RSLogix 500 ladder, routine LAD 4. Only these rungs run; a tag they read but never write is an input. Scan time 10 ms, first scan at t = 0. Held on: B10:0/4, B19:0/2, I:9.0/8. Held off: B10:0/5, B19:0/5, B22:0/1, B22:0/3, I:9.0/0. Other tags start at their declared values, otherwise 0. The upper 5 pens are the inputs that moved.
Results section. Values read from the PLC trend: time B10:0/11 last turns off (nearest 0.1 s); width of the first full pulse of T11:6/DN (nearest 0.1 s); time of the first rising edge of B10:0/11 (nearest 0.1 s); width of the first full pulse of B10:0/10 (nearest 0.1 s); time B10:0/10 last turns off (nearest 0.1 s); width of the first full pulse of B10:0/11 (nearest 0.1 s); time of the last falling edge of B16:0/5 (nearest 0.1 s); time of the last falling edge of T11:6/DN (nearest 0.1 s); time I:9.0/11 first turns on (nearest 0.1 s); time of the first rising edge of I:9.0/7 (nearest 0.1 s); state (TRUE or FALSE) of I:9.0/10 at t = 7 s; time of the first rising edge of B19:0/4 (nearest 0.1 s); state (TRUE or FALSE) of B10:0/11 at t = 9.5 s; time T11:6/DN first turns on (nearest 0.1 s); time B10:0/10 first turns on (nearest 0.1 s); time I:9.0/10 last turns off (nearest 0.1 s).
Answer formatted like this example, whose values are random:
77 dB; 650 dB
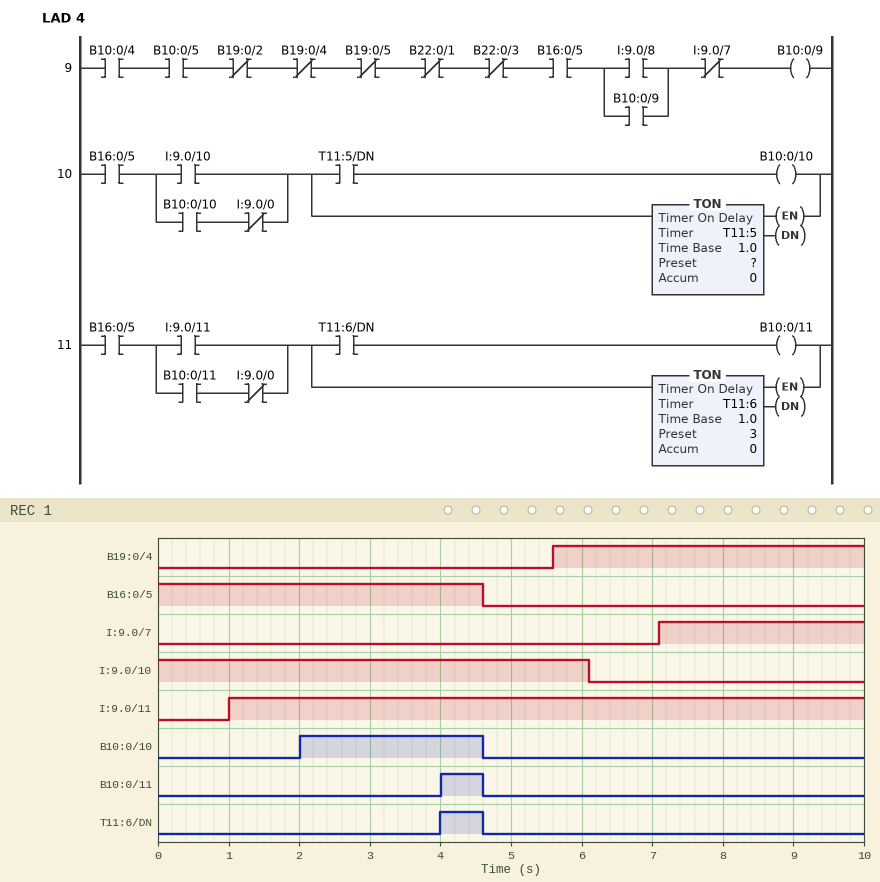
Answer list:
4.6 s; 0.6 s; 4.0 s; 2.6 s; 4.6 s; 0.6 s; 4.6 s; 4.6 s; 1.0 s; 7.1 s; FALSE; 5.6 s; FALSE; 4.0 s; 2.0 s; 6.1 s
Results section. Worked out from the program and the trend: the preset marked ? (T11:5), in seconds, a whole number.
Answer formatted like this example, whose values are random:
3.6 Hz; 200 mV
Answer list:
2 s
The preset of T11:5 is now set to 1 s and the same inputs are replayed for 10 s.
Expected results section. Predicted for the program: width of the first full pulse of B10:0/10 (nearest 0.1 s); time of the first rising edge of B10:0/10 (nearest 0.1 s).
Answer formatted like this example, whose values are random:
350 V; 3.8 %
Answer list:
3.6 s; 1.0 s
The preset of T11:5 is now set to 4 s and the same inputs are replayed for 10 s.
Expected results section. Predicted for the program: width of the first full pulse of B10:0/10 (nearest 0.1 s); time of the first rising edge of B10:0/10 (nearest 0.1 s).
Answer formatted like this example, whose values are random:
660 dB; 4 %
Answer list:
0.6 s; 4.0 s
